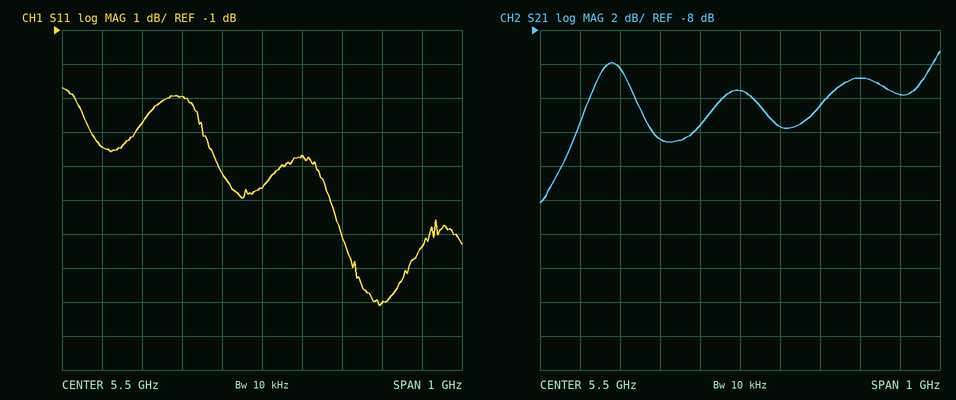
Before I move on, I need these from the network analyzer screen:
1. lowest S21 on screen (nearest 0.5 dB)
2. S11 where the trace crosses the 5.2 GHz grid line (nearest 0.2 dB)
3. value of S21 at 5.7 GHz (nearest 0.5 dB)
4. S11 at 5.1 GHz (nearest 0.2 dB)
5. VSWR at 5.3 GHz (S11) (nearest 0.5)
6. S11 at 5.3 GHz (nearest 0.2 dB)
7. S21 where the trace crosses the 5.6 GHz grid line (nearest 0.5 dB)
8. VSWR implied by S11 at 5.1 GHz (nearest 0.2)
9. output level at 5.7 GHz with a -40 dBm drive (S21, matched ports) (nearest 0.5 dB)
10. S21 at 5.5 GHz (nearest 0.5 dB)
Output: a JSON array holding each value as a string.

["-18.0 dB", "-3.8 dB", "-12.5 dB", "-4.4 dB", "6.0", "-3.0 dB", "-13.5 dB", "4.0", "-52.5 dBm", "-11.5 dB"]
